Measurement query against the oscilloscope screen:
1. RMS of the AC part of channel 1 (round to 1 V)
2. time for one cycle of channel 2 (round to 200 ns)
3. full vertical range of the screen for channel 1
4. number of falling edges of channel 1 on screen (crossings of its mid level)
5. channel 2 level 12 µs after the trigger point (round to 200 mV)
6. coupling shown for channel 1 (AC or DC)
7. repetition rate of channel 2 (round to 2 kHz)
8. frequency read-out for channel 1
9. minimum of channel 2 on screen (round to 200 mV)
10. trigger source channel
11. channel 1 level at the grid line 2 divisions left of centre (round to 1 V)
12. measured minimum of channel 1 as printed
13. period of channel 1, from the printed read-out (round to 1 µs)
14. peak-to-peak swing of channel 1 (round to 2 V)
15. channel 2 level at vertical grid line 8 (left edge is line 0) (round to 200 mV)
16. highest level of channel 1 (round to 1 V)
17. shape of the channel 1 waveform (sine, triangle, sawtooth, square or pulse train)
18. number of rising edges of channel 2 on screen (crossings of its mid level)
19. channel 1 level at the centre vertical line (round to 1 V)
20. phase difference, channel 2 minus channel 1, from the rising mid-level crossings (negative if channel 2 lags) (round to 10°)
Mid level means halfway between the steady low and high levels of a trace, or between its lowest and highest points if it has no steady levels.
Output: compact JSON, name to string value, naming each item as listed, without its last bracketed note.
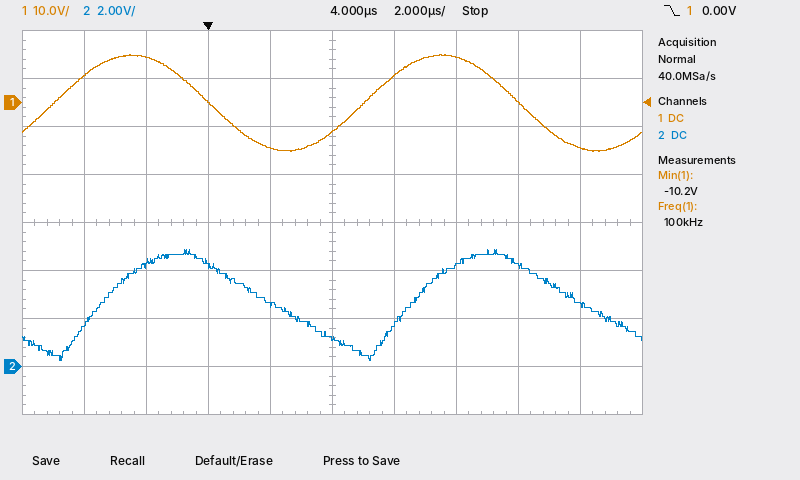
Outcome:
{"RMS of the AC part of channel 1": "7 V", "time for one cycle of channel 2": "10.0 µs", "full vertical range of the screen for channel 1": "80 V", "number of falling edges of channel 1 on screen": "2", "channel 2 level 12 µs after the trigger point": "2.6 V", "coupling shown for channel 1": "DC", "repetition rate of channel 2": "100 kHz", "frequency read-out for channel 1": "100 kHz", "minimum of channel 2 on screen": "200 mV", "trigger source channel": "channel 1", "channel 1 level at the grid line 2 divisions left of centre": "0 V", "measured minimum of channel 1 as printed": "-10.2 V", "period of channel 1, from the printed read-out": "10 µs", "peak-to-peak swing of channel 1": "20 V", "channel 2 level at vertical grid line 8 (left edge is line 0)": "4.2 V", "highest level of channel 1": "10 V", "shape of the channel 1 waveform": "sine", "number of rising edges of channel 2 on screen": "2", "channel 1 level at the centre vertical line": "-6 V", "phase difference, channel 2 minus channel 1, from the rising mid-level crossings (negative if channel 2 lags)": "-50°"}
